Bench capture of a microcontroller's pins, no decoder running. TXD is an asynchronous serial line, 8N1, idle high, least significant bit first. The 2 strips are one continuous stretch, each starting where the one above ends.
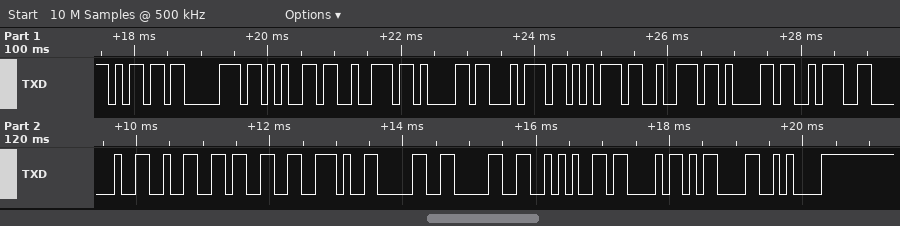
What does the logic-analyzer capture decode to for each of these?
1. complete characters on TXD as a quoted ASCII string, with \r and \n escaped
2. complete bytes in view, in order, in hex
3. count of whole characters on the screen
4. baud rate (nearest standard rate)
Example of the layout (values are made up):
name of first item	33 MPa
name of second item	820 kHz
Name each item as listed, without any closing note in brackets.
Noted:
complete characters on TXD as a quoted ASCII string, with \r and \n escaped	"mperatura: 23.00*C\r\n"
complete bytes in view, in order, in hex	0x6D 0x70 0x65 0x72 0x61 0x74 0x75 0x72 0x61 0x3A 0x20 0x32 0x33 0x2E 0x30 0x30 0x2A 0x43 0x0D 0x0A
count of whole characters on the screen	20
baud rate	9600 baud
